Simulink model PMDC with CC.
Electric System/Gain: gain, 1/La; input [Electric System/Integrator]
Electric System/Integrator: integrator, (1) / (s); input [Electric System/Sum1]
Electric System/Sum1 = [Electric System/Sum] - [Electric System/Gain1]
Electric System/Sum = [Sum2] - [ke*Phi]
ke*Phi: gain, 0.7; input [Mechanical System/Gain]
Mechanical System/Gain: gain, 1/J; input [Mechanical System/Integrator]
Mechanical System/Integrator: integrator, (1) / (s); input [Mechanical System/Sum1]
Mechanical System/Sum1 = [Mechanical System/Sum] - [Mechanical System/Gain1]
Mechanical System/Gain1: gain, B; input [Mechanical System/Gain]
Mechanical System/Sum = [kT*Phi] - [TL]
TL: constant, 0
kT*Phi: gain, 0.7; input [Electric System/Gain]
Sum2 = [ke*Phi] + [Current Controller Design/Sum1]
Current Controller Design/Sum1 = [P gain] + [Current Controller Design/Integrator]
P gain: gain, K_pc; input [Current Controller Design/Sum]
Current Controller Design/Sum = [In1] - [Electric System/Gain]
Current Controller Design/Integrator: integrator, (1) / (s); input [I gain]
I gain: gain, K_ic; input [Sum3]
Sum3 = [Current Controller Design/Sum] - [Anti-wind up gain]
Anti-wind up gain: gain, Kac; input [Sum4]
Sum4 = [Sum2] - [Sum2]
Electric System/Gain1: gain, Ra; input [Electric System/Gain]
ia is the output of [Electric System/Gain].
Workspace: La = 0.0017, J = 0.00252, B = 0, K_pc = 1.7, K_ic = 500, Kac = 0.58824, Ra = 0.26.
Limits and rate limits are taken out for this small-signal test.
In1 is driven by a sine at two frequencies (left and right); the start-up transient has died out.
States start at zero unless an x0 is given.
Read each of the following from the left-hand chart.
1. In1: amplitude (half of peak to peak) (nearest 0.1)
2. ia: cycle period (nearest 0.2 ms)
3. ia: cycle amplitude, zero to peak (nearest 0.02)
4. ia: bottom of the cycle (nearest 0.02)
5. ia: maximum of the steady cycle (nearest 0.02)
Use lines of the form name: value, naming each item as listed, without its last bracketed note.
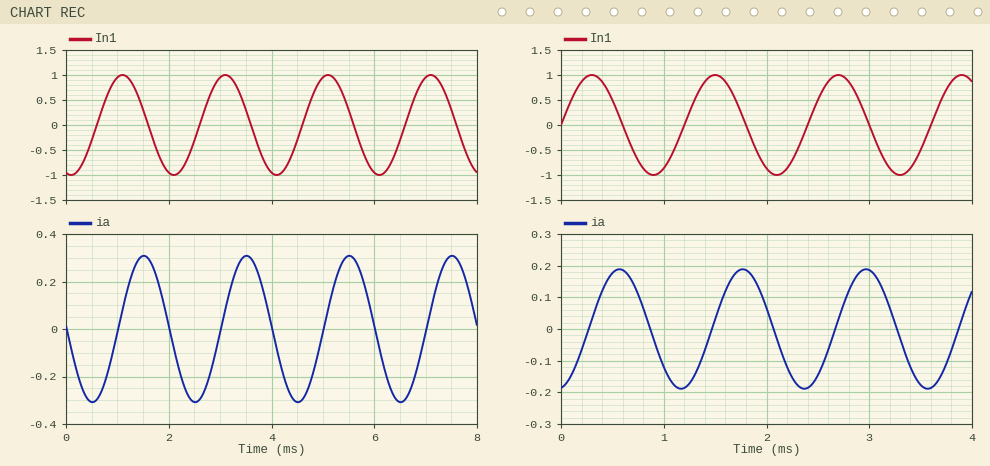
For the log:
In1: amplitude (half of peak to peak): 1.0
ia: cycle period: 2.0 ms
ia: cycle amplitude, zero to peak: 0.30
ia: bottom of the cycle: -0.30
ia: maximum of the steady cycle: 0.30
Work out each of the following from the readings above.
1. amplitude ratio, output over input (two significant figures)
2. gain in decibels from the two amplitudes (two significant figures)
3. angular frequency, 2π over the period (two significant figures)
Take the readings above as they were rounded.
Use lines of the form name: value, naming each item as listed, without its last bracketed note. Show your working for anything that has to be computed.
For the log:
amplitude ratio, output over input: 0.3 / 1 = 0.30
gain in decibels from the two amplitudes: 20 log10(0.3 / 1) = -10 dB
angular frequency, 2π over the period: 2π / 2 = 3.1 rad/ms
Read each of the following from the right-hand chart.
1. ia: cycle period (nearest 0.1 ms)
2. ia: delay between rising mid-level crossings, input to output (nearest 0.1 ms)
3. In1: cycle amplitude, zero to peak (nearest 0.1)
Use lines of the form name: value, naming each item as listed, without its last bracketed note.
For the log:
ia: cycle period: 1.2 ms
ia: delay between rising mid-level crossings, input to output: 0.3 ms
In1: cycle amplitude, zero to peak: 1.0
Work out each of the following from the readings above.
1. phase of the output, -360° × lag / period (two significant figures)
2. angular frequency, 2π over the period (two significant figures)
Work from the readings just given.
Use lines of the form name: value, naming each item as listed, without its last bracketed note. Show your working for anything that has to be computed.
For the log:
phase of the output, -360° × lag / period: -360 × 0.3 / 1.2 = -90°
angular frequency, 2π over the period: 2π / 1.2 = 5.2 rad/ms
